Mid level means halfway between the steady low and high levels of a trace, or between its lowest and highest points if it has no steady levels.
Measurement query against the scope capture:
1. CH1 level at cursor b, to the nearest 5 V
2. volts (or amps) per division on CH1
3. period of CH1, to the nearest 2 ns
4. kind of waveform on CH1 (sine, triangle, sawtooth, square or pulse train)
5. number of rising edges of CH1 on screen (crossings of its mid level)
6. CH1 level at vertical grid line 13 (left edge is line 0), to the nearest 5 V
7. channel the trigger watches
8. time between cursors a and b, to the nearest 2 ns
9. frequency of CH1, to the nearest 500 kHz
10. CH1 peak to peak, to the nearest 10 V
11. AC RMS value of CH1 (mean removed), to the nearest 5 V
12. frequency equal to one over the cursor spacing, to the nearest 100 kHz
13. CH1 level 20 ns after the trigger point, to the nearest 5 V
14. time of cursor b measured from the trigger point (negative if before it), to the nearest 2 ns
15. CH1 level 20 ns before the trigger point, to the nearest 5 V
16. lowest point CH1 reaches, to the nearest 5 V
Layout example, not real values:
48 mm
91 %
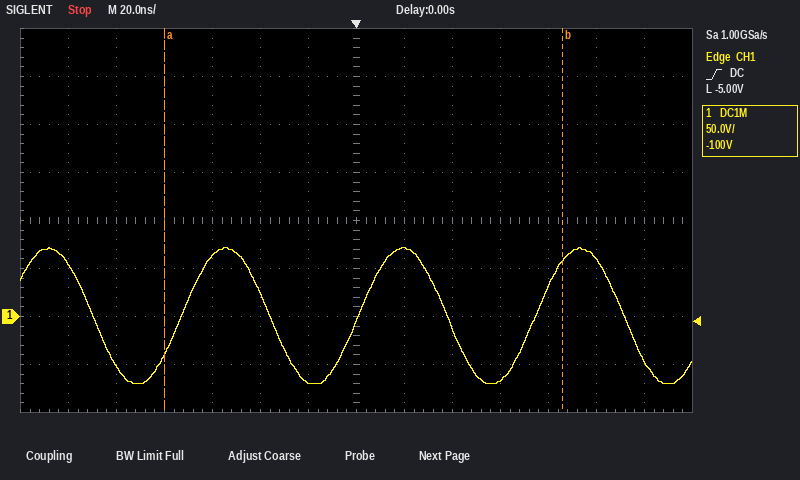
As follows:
60 V
50 V
74 ns
sine
3
-45 V
CH1
166 ns
13.5 MHz
140 V
50 V
6.0 MHz
70 V
+86 ns
-70 V
-70 V
